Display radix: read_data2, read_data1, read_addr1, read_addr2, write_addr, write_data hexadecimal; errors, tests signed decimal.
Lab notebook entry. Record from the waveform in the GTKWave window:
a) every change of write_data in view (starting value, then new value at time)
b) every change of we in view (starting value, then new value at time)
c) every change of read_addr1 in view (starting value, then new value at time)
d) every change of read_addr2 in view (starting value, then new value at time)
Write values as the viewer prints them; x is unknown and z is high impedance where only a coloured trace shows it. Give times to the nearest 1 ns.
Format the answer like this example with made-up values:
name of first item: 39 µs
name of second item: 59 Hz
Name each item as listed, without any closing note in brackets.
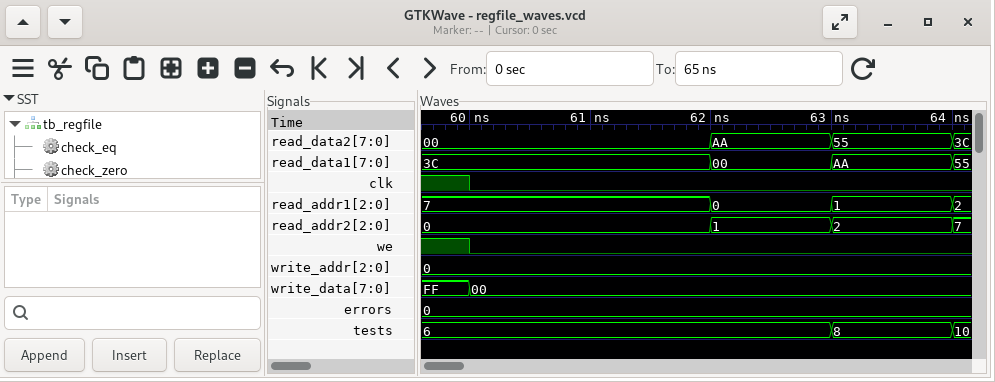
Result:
every change of write_data in view: FF, 00 at 60 ns
every change of we in view: 1, 0 at 60 ns
every change of read_addr1 in view: 7, 0 at 62 ns, 1 at 63 ns, 2 at 64 ns
every change of read_addr2 in view: 0, 1 at 62 ns, 2 at 63 ns, 7 at 64 ns
